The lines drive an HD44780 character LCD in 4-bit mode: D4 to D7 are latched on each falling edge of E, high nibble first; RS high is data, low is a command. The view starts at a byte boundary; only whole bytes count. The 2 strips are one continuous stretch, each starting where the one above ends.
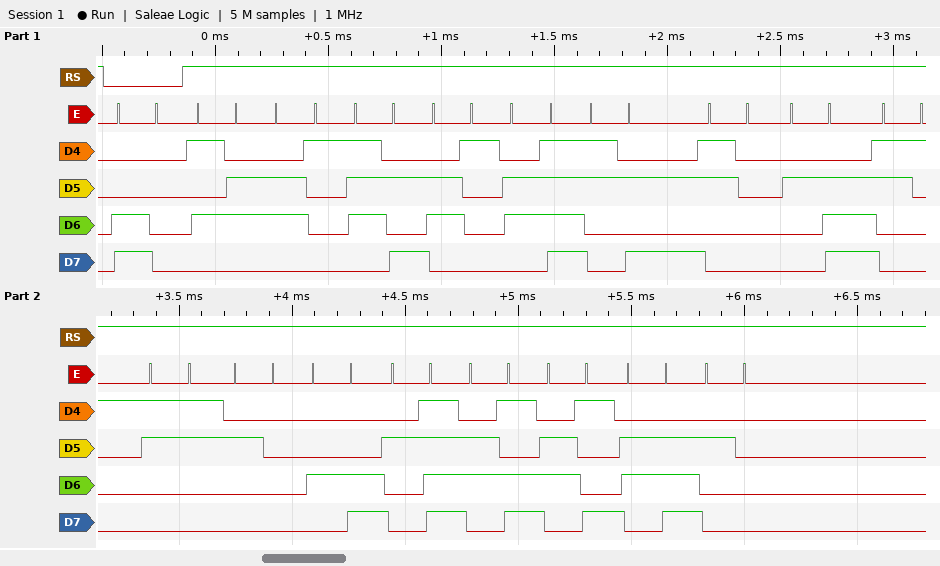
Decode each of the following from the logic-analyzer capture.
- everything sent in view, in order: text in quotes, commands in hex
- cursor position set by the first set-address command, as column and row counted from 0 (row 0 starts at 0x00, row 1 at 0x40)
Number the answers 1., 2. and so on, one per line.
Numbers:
1. 0xC0 "Vazao:0.13 L/min "
2. column 0, row 1
